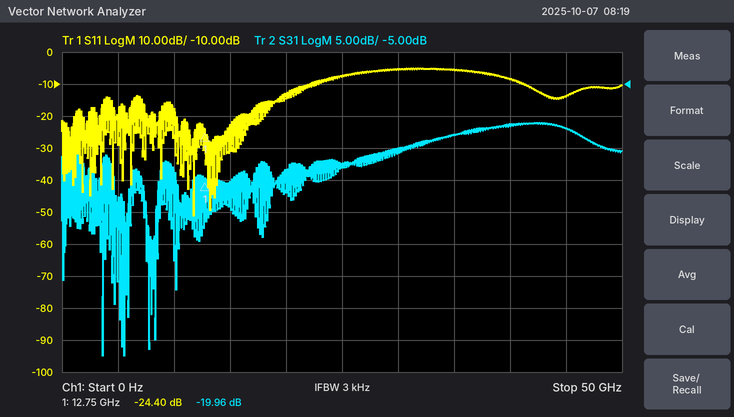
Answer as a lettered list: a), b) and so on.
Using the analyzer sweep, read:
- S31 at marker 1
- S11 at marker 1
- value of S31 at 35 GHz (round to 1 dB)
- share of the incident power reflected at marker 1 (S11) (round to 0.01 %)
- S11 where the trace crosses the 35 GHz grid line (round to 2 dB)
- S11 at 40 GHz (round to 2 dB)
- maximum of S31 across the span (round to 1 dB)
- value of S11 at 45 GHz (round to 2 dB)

a) -19.96 dB
b) -24.40 dB
c) -13 dB
d) 0.36 %
e) -6 dB
f) -8 dB
g) -11 dB
h) -14 dB
